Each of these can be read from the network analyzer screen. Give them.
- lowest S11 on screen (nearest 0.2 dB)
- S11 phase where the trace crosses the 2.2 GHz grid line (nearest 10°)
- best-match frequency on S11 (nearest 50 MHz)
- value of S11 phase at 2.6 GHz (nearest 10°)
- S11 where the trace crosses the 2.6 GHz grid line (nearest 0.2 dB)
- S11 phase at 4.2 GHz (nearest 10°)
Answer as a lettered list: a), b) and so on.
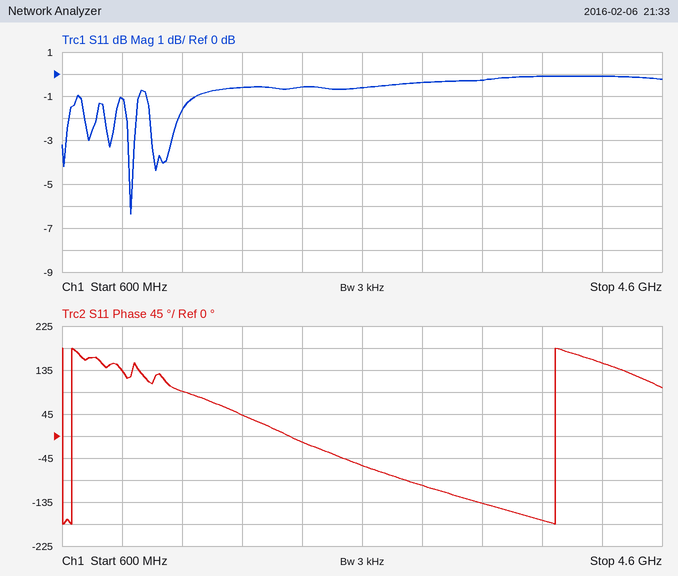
a) -6.4 dB
b) -10°
c) 1.05 GHz
d) -60°
e) -0.6 dB
f) 150°
